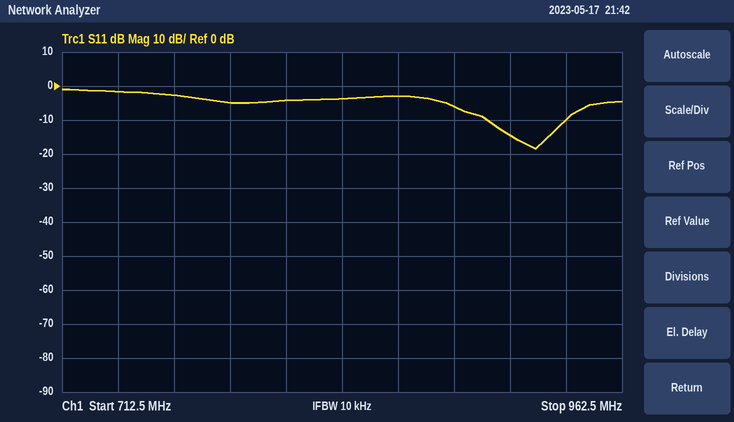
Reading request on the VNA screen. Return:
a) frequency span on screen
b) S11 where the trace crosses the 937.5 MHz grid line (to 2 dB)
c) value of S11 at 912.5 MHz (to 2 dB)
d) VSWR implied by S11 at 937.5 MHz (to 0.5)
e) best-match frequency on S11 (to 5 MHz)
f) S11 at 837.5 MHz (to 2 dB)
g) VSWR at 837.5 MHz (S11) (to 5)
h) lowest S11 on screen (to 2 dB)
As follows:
250 MHz
-10 dB
-14 dB
2.0
925 MHz
-4 dB
5
-18 dB
